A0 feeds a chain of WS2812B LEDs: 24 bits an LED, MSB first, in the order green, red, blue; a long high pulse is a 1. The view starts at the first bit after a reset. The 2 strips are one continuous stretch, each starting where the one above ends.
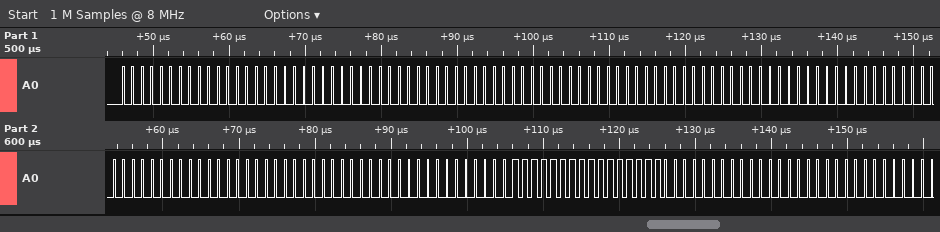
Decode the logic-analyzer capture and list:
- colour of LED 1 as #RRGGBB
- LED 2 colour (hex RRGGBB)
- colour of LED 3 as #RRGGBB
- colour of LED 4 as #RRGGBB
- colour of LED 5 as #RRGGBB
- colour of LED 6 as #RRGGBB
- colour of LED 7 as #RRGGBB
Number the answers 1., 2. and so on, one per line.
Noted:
1. #000000
2. #000000
3. #000000
4. #000000
5. #000000
6. #FF00FF
7. #000000
